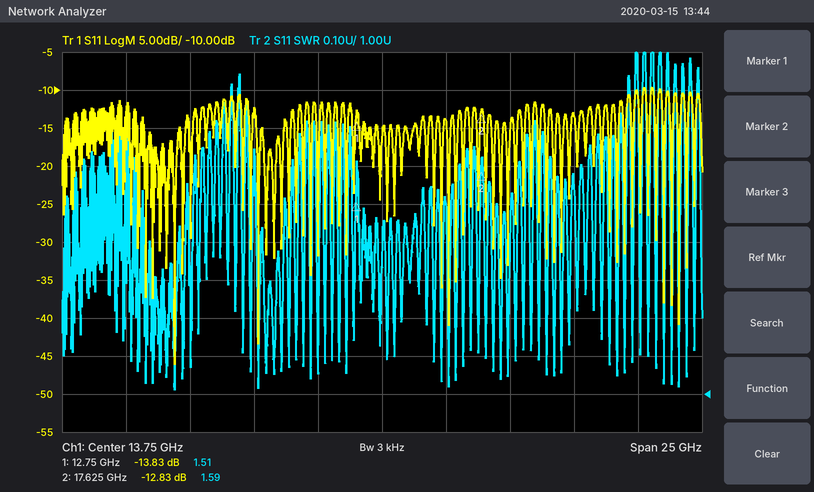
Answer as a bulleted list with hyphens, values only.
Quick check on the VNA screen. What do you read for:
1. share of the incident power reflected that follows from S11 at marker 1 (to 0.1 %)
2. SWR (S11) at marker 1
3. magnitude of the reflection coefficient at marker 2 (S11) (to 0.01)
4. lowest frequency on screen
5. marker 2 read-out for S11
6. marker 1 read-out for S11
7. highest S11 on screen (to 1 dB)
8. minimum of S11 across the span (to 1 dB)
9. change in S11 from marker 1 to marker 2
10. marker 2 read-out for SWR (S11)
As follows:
- 4.1 %
- 1.51
- 0.23
- 1.25 GHz
- -12.83 dB
- -13.83 dB
- -10 dB
- -46 dB
- 1.00 dB
- 1.59
